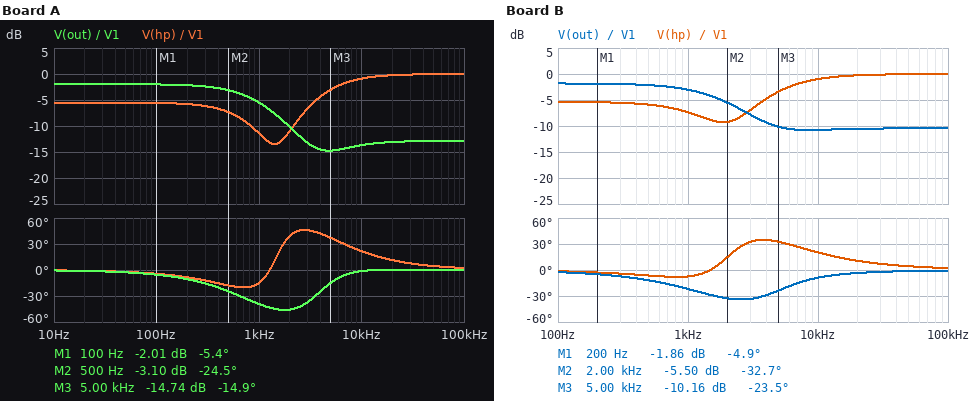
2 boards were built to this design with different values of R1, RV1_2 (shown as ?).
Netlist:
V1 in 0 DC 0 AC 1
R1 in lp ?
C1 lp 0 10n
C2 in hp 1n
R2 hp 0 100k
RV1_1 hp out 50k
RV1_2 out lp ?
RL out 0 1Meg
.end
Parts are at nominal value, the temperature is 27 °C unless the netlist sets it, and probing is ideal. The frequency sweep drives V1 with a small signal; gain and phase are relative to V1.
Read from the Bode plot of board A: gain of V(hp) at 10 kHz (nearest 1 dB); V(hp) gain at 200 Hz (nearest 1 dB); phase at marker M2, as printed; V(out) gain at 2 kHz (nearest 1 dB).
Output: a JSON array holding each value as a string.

["-1 dB", "-6 dB", "-24.5 deg", "-10 dB"]
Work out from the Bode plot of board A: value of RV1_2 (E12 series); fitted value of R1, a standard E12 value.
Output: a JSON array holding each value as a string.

["15 kΩ", "18 kΩ"]
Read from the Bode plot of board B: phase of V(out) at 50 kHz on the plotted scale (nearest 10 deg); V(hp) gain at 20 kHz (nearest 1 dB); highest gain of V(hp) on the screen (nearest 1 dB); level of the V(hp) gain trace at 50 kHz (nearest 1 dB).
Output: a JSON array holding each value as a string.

["0 deg", "0 dB", "0 dB", "0 dB"]
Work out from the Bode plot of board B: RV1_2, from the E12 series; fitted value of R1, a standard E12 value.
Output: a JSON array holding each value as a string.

["22 kΩ", "8.2 kΩ"]
